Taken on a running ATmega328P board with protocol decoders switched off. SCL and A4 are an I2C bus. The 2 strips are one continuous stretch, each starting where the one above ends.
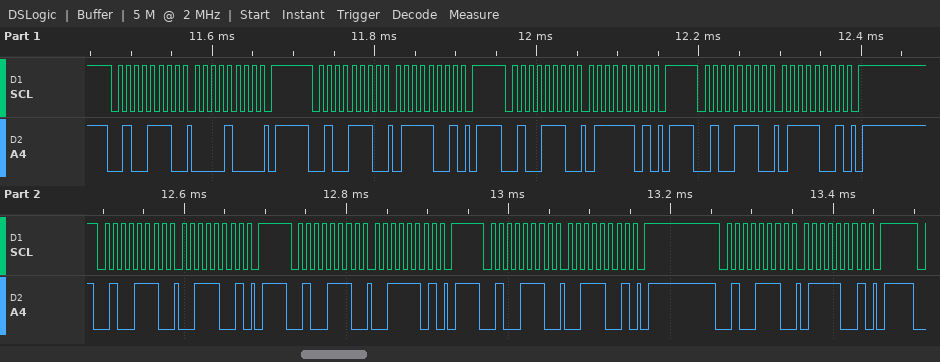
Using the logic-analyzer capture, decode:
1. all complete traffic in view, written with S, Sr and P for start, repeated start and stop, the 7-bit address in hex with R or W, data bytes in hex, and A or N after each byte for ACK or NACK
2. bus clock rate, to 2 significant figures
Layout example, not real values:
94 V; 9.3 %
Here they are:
S 27W A 08 A P S 27W A 79 A P S 27W A 7D A P S 27W A 79 A P S 27W A 39 A P S 27W A 3D A P S 27W A 39 A P S 27W A 79 A P; 100 kHz
